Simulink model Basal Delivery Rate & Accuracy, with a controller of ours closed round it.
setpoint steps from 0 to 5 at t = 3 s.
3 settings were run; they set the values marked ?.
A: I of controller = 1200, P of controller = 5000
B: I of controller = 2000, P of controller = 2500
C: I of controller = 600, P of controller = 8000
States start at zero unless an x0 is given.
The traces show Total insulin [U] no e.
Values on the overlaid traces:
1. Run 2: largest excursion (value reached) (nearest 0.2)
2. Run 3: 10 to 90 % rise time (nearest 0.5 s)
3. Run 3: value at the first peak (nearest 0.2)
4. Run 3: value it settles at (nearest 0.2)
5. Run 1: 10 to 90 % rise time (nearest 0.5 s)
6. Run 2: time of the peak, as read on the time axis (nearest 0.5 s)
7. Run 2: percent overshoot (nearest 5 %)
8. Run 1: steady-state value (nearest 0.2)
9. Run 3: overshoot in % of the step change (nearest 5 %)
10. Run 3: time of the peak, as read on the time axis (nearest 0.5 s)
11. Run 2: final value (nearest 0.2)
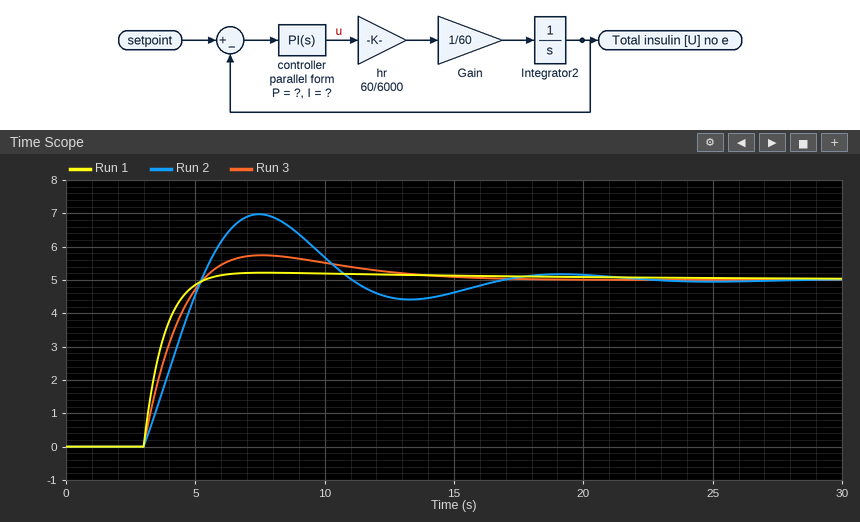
7.0
1.5 s
5.8
5.0
1.5 s
7.5 s
40 %
5.0
15 %
7.5 s
5.0
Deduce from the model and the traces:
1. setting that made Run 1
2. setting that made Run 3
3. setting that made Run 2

C
A
B
